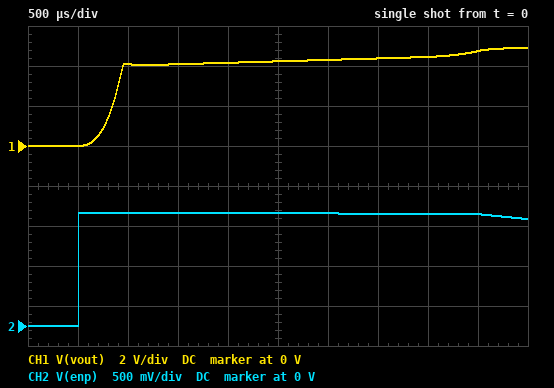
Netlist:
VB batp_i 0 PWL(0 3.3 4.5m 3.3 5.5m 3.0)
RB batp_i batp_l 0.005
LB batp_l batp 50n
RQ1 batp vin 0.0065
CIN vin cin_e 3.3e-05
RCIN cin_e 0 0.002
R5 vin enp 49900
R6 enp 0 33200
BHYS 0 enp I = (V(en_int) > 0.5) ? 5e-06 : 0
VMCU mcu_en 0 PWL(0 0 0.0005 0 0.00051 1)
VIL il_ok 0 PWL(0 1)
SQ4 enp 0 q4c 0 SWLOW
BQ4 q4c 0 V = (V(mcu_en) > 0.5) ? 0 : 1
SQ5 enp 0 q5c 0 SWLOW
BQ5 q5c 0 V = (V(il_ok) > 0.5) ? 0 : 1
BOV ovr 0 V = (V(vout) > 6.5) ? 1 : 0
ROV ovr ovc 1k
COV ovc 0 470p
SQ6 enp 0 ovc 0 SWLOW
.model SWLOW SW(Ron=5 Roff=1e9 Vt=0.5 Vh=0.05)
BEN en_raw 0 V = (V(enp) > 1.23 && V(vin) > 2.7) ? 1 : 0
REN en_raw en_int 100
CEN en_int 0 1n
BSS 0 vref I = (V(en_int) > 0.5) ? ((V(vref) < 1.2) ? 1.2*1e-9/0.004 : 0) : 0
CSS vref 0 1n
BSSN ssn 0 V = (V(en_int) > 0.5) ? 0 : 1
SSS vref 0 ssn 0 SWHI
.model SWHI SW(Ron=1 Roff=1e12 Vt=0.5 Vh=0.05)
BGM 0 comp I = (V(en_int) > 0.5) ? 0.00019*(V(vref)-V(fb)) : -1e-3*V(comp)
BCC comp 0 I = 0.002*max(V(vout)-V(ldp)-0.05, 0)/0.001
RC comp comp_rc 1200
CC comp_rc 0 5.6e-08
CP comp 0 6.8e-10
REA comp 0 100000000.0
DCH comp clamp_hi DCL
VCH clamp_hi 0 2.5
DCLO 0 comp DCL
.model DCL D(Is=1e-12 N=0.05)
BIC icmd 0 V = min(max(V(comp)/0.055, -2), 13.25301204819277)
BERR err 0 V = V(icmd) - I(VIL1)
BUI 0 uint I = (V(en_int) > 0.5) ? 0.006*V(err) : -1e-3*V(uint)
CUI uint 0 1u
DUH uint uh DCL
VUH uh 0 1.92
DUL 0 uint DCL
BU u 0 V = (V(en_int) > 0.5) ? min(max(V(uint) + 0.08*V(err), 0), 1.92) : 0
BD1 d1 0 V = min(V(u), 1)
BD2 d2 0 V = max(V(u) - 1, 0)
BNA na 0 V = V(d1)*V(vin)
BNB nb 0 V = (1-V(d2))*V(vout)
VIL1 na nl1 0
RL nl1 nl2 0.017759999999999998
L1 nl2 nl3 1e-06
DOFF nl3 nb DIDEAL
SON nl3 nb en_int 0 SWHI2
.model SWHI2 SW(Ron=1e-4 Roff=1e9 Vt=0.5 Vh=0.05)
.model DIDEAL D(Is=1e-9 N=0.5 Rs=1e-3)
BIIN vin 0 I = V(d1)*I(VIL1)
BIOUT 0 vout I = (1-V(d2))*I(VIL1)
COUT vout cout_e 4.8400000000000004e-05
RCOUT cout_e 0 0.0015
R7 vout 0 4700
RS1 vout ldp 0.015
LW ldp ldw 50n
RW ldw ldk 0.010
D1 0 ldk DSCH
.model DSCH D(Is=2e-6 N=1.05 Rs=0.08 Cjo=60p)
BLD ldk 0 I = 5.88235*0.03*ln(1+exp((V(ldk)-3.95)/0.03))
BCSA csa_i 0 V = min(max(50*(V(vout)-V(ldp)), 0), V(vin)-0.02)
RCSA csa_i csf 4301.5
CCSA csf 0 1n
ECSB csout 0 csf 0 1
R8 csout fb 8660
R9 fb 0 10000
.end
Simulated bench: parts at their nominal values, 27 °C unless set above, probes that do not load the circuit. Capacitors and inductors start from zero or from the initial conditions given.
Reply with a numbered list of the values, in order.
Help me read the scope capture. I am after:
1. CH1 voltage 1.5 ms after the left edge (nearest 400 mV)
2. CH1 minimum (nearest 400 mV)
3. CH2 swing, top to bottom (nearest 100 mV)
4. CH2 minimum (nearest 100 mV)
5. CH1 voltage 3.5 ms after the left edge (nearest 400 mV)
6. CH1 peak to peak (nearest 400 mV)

1. 4.0 V
2. 0 V
3. 1.4 V
4. 0 V
5. 4.4 V
6. 4.8 V
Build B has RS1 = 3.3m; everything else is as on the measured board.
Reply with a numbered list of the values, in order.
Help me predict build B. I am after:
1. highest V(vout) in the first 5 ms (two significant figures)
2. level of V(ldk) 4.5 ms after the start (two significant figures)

1. 6.5 V
2. 4.4 V
